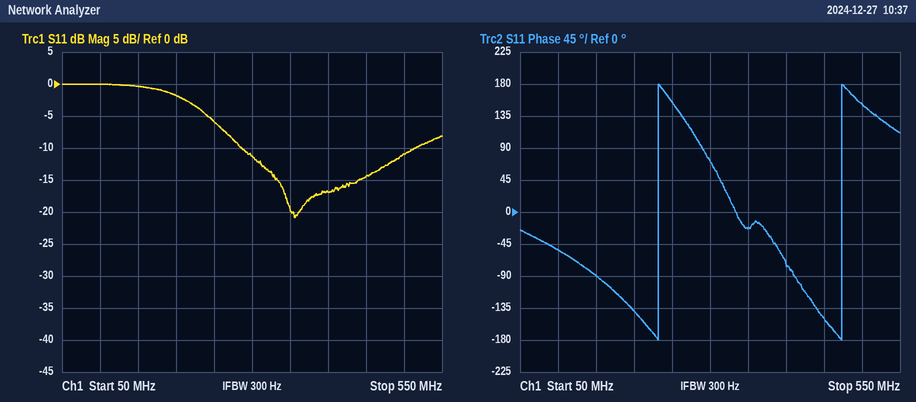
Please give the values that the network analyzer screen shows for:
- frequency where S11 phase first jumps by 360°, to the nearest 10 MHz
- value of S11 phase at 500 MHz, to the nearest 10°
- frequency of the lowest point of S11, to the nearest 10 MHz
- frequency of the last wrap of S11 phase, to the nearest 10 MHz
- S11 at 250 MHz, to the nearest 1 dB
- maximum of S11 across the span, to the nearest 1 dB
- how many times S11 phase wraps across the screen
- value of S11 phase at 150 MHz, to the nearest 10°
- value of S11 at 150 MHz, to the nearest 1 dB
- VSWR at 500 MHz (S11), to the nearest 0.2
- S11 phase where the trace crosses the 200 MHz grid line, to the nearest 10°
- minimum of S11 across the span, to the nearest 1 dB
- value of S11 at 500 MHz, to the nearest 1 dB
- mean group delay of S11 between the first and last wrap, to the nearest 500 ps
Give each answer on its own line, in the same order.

230 MHz
150°
360 MHz
470 MHz
-6 dB
0 dB
2
-90°
0 dB
1.8
-140°
-21 dB
-11 dB
4.0 ns
